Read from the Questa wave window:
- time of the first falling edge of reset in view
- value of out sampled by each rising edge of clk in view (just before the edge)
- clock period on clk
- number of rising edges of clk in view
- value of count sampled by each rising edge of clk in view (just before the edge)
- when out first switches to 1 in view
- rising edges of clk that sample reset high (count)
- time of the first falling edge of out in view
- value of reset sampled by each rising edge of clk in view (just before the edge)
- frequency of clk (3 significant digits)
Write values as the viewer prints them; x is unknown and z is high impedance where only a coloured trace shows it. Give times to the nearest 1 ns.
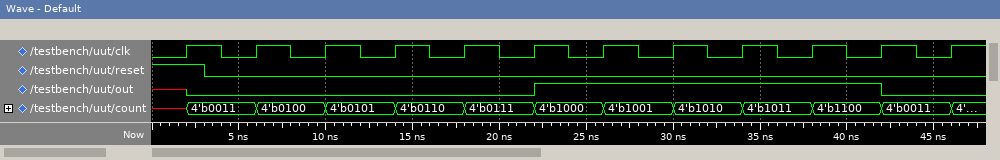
3 ns
x 0 0 0 0 0 1 1 1 1 1 0
4 ns
12
x, 4'b0011, 4'b0100, 4'b0101, 4'b0110, 4'b0111, 4'b1000, 4'b1001, 4'b1010, 4'b1011, 4'b1100, 4'b0011
22 ns
1
42 ns
1 0 0 0 0 0 0 0 0 0 0 0
250 MHz
